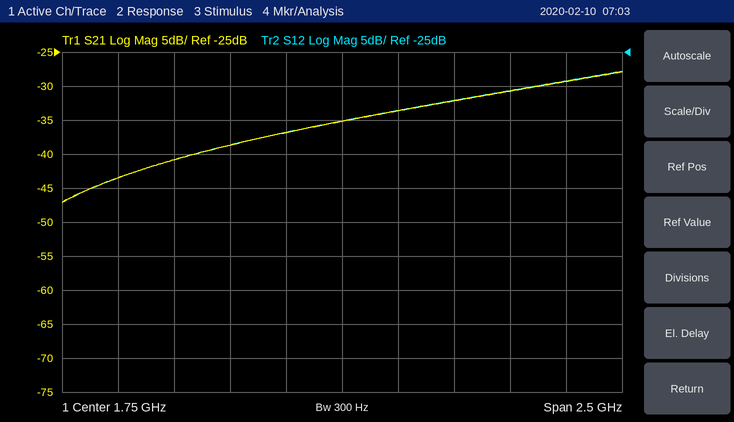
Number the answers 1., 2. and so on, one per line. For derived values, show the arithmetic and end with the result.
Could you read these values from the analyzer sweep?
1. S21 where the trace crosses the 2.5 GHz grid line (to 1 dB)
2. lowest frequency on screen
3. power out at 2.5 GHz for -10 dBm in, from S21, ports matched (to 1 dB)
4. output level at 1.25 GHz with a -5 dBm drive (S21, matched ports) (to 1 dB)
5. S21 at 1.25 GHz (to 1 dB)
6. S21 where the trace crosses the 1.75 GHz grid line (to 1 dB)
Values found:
1. -31 dB
2. 500 MHz
3. -10 dBm + (-31 dB) = -41 dBm
4. -5 dBm + (-39 dB) = -44 dBm
5. -39 dB
6. -35 dB
